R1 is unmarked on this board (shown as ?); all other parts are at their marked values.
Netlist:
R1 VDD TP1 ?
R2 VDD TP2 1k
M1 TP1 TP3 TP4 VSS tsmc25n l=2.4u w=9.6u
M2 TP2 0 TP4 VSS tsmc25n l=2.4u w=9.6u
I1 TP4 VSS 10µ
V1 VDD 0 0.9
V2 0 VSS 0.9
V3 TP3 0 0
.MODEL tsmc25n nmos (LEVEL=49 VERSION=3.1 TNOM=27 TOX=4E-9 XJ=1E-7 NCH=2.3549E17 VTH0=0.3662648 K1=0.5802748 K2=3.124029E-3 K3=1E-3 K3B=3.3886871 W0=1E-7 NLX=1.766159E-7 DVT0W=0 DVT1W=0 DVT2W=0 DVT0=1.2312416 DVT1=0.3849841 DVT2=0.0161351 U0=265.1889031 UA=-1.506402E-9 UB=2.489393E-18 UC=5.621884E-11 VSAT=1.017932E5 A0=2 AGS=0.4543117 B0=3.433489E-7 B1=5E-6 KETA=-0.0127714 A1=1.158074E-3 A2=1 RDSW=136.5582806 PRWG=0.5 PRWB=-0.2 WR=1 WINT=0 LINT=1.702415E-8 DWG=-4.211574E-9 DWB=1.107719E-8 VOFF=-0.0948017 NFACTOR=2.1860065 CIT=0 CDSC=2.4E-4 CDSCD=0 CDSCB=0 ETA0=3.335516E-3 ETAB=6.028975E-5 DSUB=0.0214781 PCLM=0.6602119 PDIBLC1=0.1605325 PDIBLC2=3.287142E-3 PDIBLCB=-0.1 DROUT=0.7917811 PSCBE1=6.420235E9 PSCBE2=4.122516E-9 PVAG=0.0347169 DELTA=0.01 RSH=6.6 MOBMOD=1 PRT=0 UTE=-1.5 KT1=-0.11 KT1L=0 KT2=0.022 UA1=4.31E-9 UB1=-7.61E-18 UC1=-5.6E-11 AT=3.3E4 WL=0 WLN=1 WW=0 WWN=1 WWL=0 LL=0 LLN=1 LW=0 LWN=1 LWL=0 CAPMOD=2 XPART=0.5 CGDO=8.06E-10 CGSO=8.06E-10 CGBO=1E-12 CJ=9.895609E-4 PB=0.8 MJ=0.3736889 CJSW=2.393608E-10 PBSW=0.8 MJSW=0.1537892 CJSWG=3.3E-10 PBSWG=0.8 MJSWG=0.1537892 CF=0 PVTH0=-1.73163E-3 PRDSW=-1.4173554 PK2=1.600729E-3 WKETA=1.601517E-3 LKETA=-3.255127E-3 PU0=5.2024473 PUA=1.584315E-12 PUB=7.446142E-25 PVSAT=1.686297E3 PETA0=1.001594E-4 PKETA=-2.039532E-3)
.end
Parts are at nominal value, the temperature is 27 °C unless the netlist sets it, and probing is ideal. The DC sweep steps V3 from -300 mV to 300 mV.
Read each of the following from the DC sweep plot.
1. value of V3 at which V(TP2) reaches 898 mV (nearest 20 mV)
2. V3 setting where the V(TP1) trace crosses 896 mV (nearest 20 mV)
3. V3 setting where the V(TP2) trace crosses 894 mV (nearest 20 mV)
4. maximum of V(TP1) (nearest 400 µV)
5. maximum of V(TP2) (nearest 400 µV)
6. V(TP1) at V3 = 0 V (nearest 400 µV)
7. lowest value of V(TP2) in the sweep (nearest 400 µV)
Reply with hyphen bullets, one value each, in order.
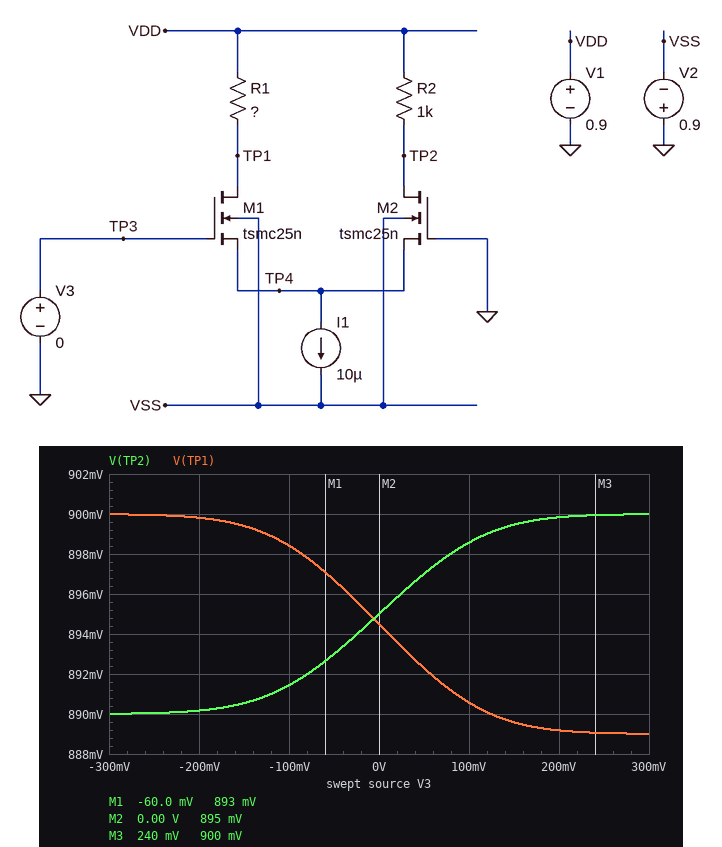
- 80 mV
- -40 mV
- -20 mV
- 900.0 mV
- 900.0 mV
- 894.4 mV
- 890.0 mV
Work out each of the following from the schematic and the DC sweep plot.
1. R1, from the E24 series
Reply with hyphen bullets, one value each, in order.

- 1.1 kΩ
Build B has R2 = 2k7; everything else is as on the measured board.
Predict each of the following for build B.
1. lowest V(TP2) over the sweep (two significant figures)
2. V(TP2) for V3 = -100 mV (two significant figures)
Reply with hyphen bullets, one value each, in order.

- 870 mV
- 880 mV
